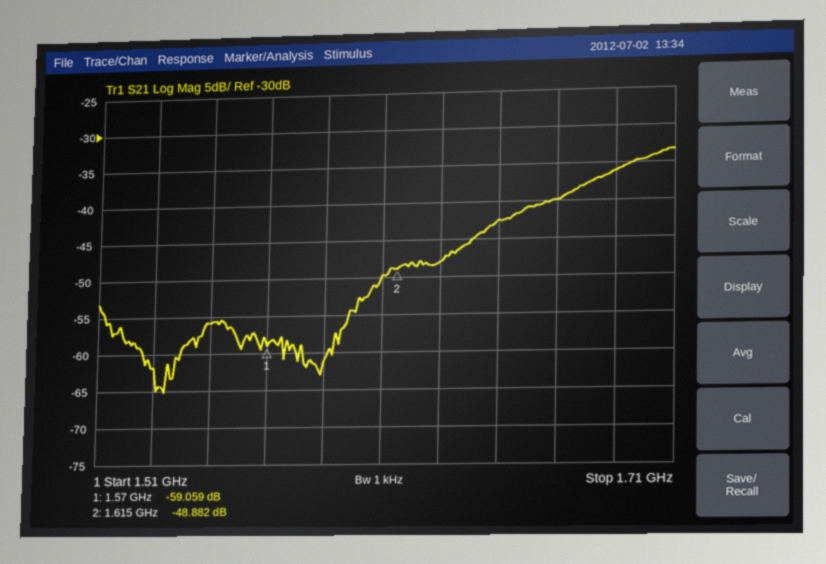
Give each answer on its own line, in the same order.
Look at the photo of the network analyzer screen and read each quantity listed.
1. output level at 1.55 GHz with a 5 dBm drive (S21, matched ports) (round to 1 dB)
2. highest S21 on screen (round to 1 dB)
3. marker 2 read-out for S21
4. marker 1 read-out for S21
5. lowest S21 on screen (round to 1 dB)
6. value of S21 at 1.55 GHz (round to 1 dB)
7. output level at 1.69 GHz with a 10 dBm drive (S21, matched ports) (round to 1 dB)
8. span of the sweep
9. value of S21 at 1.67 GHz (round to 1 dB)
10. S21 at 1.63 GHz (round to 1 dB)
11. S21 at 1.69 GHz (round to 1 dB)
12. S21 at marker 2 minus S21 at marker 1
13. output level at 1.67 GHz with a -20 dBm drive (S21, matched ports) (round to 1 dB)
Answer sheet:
-51 dBm
-33 dB
-48.882 dB
-59.059 dB
-65 dB
-56 dB
-26 dBm
200 MHz
-40 dB
-48 dB
-36 dB
10.177 dB
-60 dBm
